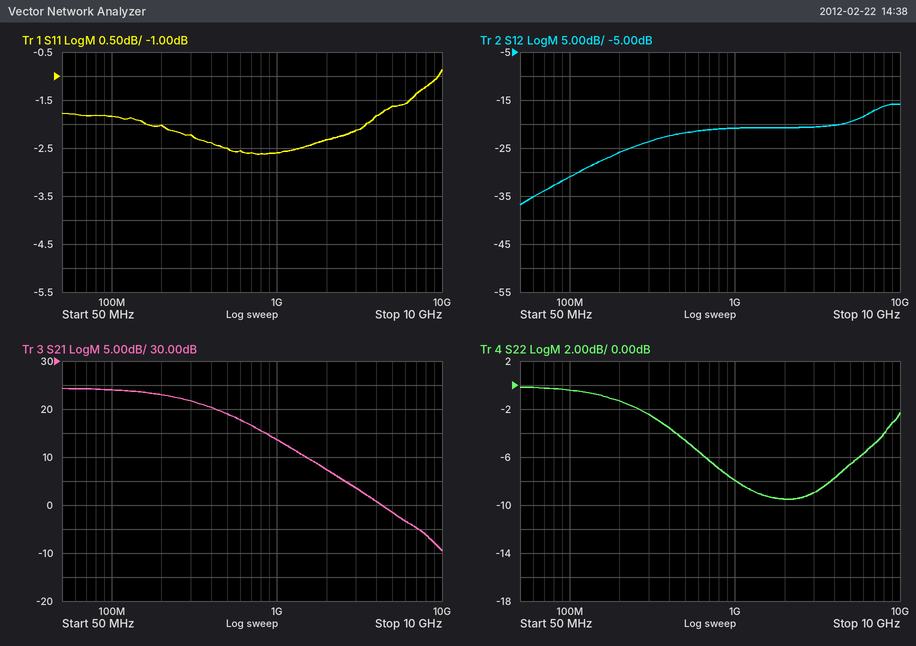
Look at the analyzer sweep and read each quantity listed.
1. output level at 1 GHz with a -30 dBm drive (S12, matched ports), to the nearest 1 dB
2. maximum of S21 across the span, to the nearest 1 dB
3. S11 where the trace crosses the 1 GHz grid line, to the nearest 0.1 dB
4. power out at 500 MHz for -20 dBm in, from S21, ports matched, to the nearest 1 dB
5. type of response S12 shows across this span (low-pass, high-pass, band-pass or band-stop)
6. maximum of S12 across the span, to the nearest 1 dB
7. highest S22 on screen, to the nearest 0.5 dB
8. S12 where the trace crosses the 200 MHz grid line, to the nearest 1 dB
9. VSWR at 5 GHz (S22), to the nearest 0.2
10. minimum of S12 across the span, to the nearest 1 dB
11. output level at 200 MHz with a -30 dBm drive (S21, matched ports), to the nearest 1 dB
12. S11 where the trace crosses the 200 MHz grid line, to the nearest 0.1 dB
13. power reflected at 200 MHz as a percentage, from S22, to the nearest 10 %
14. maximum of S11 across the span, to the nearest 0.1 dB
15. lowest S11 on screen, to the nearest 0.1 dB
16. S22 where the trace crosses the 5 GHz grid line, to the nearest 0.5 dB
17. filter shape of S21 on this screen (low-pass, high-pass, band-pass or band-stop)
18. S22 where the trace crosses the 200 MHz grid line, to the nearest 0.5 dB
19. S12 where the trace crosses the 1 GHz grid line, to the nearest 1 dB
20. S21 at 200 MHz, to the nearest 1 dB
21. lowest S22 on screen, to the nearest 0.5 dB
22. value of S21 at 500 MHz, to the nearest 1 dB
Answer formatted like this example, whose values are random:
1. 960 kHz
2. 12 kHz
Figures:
1. -51 dBm
2. 24 dB
3. -2.6 dB
4. -1 dBm
5. high-pass
6. -16 dB
7. 0.0 dB
8. -26 dB
9. 2.8
10. -37 dB
11. -7 dBm
12. -2.0 dB
13. 70 %
14. -0.9 dB
15. -2.6 dB
16. -6.5 dB
17. low-pass
18. -1.5 dB
19. -21 dB
20. 23 dB
21. -9.5 dB
22. 19 dB
